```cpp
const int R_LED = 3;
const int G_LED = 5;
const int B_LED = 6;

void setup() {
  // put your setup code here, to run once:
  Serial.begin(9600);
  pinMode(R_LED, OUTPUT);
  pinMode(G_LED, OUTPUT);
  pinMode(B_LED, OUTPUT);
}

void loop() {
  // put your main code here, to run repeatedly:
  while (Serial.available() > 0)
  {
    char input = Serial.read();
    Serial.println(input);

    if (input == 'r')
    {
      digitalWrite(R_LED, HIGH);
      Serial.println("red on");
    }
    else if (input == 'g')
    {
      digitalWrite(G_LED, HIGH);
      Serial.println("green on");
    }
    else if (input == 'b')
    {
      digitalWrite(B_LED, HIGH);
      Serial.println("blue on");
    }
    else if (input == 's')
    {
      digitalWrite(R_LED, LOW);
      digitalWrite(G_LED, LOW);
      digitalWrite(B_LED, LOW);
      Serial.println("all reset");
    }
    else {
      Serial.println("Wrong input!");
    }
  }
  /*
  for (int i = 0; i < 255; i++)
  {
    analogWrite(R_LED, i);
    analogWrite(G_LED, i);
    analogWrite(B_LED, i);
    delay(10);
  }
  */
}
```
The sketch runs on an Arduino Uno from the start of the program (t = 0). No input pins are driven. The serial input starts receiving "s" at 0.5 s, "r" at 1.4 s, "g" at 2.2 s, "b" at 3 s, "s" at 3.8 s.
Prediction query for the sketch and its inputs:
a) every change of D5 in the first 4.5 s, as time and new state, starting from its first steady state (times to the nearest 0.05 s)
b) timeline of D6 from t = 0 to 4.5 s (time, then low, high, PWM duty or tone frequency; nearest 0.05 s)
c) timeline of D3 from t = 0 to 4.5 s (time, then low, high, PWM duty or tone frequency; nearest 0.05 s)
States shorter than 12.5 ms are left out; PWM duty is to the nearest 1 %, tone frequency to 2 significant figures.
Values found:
0 s low; 2.2 s high; 3.8 s low
0 s low; 3 s high; 3.8 s low
0 s low; 1.4 s high; 3.8 s low
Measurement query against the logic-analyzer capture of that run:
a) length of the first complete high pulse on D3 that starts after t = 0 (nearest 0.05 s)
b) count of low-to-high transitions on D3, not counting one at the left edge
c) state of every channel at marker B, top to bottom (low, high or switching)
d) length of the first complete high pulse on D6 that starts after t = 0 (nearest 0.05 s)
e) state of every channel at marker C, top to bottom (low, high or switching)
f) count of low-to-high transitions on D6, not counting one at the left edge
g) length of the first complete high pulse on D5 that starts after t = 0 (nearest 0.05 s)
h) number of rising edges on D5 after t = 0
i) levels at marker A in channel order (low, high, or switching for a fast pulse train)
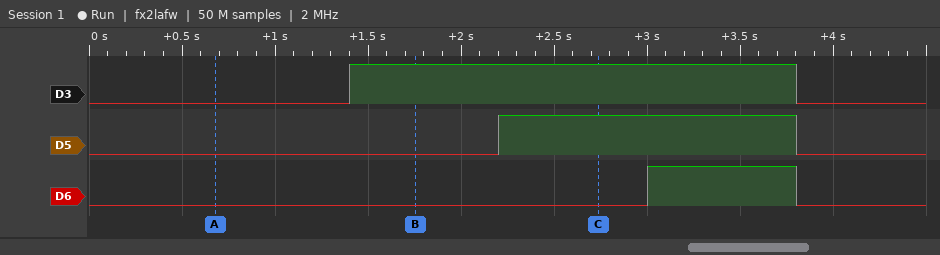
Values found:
2.40 s
1
D3 high, D5 low, D6 low
0.80 s
D3 high, D5 high, D6 low
1
1.60 s
1
D3 low, D5 low, D6 low
